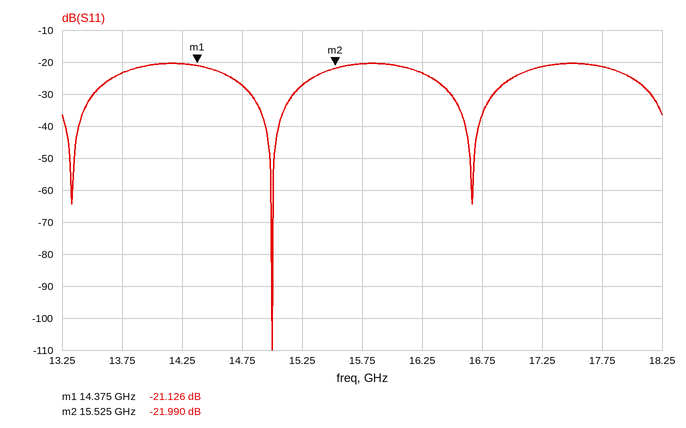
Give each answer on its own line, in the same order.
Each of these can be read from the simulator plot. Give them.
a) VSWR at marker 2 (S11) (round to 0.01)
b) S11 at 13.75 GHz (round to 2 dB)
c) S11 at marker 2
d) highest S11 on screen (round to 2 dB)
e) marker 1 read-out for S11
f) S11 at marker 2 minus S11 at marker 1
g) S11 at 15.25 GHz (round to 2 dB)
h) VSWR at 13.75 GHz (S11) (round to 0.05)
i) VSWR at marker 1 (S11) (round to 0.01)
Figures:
1.17
-24 dB
-21.990 dB
-20 dB
-21.126 dB
-0.864 dB
-28 dB
1.15
1.19
